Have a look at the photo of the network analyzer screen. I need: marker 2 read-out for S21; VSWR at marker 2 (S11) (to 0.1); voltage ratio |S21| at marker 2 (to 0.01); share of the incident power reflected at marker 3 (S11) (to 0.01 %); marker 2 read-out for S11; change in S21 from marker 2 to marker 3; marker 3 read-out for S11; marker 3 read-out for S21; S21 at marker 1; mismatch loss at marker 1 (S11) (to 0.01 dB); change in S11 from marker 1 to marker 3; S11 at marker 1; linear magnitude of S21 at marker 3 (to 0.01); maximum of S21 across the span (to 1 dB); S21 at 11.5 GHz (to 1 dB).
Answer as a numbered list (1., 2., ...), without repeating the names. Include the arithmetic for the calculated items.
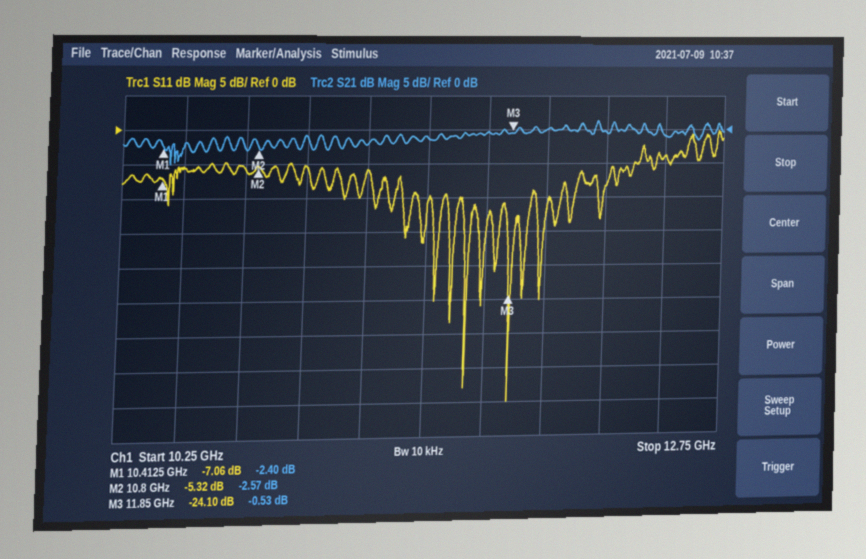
1. -2.57 dB
2. (1 + 0.5420)/(1 − 0.5420) ≈ 3.4
3. 10^(-2.57/20) ≈ 0.74
4. 10^(-24.1/10) ≈ 0.39 %
5. -5.32 dB
6. -0.53 − (-2.57) = 2.04 dB
7. -24.10 dB
8. -0.53 dB
9. -2.40 dB
10. −10 log10(1 − 10^(-7.06/10)) ≈ 0.95 dB
11. -24.1 − (-7.06) = -17.04 dB
12. -7.06 dB
13. 10^(-0.53/20) ≈ 0.94
14. 1 dB
15. -1 dB
